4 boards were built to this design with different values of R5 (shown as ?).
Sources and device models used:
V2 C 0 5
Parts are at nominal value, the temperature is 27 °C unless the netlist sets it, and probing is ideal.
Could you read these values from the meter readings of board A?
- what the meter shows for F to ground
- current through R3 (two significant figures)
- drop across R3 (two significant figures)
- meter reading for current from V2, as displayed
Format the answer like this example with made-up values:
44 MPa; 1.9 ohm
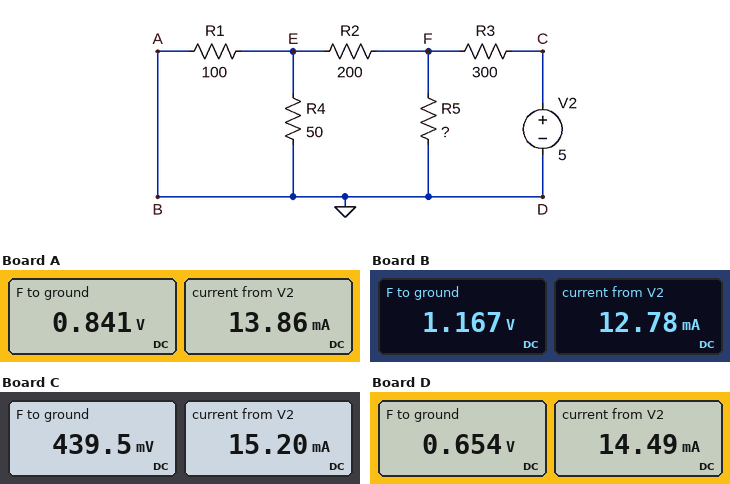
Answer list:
0.841 V; 14 mA; 4.2 V; 13.86 mA
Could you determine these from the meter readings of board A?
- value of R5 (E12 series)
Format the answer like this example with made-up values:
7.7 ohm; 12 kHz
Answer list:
82 Ω
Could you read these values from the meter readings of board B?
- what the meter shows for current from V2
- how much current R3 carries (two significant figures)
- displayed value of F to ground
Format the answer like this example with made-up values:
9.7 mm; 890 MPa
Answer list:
12.78 mA; 13 mA; 1.167 V
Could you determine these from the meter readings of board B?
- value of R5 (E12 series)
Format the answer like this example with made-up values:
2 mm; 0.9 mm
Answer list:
150 Ω
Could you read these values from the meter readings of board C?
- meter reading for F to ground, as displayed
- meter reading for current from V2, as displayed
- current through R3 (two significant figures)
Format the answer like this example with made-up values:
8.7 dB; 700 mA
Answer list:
439.5 mV; 15.20 mA; 15 mA
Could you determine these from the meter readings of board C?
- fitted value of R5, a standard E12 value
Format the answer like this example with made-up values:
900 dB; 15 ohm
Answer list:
33 Ω
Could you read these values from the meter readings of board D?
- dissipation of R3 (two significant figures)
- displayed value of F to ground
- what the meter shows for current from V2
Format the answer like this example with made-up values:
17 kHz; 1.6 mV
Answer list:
63 mW; 0.654 V; 14.49 mA
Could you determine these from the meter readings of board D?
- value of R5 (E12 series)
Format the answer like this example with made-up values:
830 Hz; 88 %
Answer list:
56 Ω
